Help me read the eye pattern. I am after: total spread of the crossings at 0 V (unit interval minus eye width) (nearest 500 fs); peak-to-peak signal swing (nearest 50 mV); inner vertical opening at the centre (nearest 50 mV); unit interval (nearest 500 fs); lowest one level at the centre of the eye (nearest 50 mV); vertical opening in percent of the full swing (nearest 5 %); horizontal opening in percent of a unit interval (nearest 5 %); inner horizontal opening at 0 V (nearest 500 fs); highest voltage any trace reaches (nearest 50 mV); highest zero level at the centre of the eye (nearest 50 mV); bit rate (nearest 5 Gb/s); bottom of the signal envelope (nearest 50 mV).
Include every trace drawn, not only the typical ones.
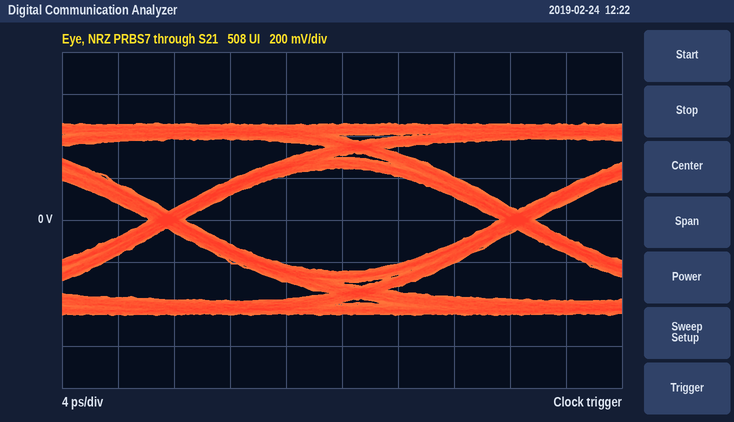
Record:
2.5 ps
900 mV
500 mV
25.0 ps
250 mV
55 %
90 %
22.5 ps
450 mV
-250 mV
40 Gb/s
-450 mV
